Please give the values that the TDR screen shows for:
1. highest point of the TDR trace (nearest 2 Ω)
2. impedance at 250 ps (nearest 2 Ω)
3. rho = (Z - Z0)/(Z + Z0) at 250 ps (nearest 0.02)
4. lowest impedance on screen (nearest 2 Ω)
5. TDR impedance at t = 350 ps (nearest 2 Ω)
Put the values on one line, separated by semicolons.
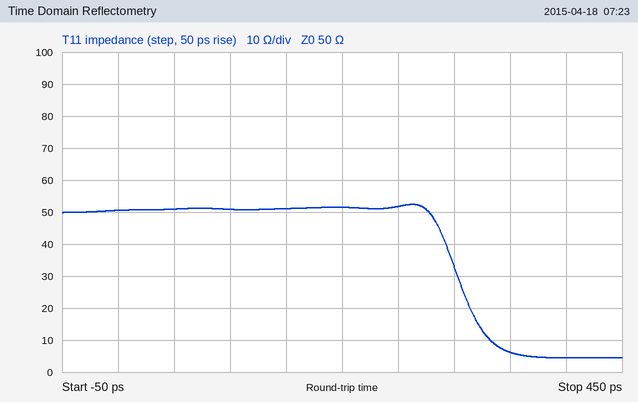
52 Ω; 52 Ω; +0.02; 4 Ω; 6 Ω
